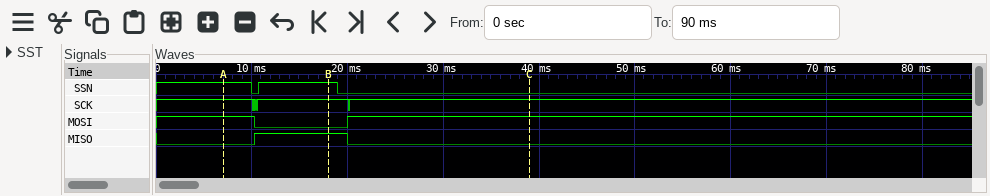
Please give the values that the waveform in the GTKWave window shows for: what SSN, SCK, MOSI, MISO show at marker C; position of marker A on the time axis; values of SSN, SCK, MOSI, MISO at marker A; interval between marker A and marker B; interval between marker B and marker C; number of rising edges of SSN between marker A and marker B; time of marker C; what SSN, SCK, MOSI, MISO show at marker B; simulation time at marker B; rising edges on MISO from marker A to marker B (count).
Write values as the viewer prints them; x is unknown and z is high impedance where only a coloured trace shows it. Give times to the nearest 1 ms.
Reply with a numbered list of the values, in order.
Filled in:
1. SSN=0, SCK=1, MOSI=1, MISO=0
2. 7 ms
3. SSN=1, SCK=1, MOSI=1, MISO=0
4. 11 ms
5. 21 ms
6. 1
7. 39 ms
8. SSN=1, SCK=1, MOSI=0, MISO=1
9. 18 ms
10. 1
